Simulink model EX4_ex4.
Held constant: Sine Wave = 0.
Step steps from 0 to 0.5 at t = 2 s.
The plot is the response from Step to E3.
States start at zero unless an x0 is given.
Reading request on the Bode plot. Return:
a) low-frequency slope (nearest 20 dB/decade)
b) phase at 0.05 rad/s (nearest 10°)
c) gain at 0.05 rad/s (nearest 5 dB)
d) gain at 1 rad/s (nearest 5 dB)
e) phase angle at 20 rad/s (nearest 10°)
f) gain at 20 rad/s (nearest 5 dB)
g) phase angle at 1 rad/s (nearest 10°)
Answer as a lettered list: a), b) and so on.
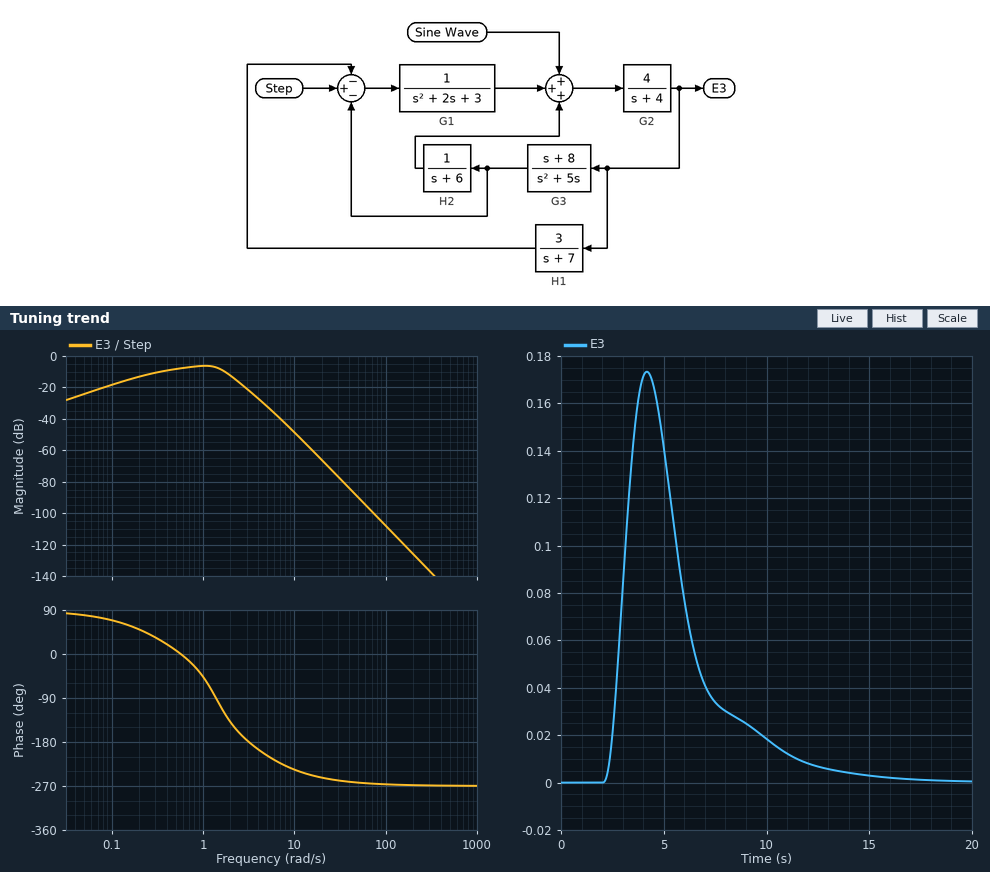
a) 20 dB/decade
b) 80°
c) -25 dB
d) -5 dB
e) -250°
f) -65 dB
g) -50°
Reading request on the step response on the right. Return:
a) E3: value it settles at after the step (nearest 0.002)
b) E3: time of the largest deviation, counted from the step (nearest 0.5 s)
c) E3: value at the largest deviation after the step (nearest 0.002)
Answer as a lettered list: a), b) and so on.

a) 0.000
b) 2.0 s
c) 0.174
